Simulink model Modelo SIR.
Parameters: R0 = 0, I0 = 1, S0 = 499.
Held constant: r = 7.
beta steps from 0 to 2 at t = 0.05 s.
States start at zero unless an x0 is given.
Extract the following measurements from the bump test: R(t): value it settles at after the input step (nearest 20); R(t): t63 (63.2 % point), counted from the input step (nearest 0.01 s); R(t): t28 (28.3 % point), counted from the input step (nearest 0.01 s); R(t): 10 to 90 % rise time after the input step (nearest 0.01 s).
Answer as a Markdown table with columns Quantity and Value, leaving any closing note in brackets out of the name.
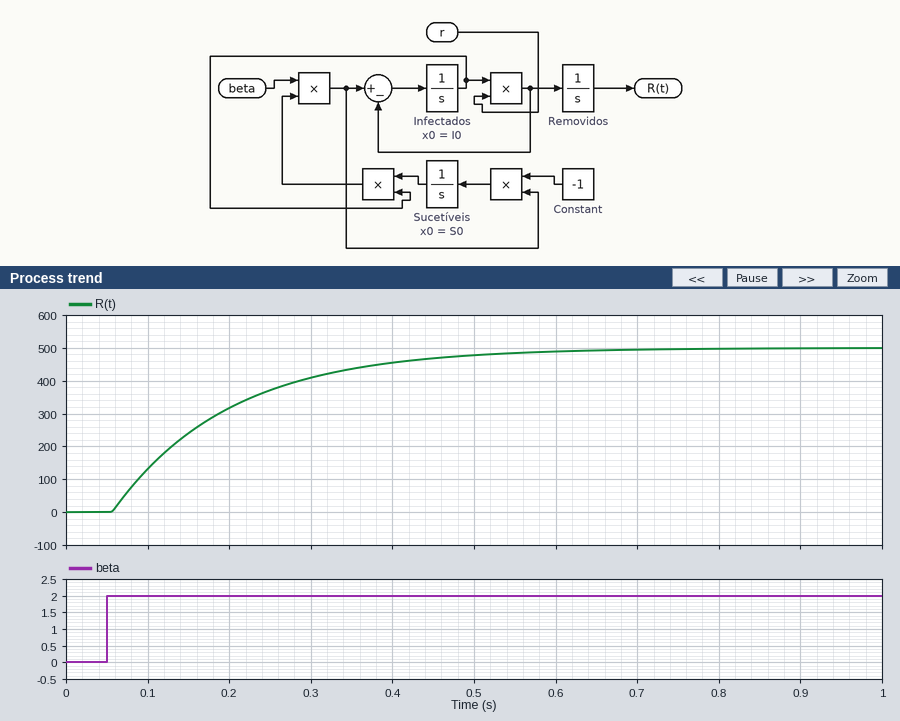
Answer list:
| Quantity | Value |
|---|---|
| R(t): value it settles at after the input step | 500 |
| R(t): t63 (63.2 % point), counted from the input step | 0.15 s |
| R(t): t28 (28.3 % point), counted from the input step | 0.05 s |
| R(t): 10 to 90 % rise time after the input step | 0.31 s |
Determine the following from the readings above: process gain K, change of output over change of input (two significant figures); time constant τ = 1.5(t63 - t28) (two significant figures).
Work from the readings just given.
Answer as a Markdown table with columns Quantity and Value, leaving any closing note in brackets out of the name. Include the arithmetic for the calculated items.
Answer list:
| Quantity | Value |
|---|---|
| process gain K, change of output over change of input | (500 - 0) / 2 = 250 |
| time constant τ = 1.5(t63 - t28) | 1.5 × (0.15 - 0.05) = 0.15 s |
